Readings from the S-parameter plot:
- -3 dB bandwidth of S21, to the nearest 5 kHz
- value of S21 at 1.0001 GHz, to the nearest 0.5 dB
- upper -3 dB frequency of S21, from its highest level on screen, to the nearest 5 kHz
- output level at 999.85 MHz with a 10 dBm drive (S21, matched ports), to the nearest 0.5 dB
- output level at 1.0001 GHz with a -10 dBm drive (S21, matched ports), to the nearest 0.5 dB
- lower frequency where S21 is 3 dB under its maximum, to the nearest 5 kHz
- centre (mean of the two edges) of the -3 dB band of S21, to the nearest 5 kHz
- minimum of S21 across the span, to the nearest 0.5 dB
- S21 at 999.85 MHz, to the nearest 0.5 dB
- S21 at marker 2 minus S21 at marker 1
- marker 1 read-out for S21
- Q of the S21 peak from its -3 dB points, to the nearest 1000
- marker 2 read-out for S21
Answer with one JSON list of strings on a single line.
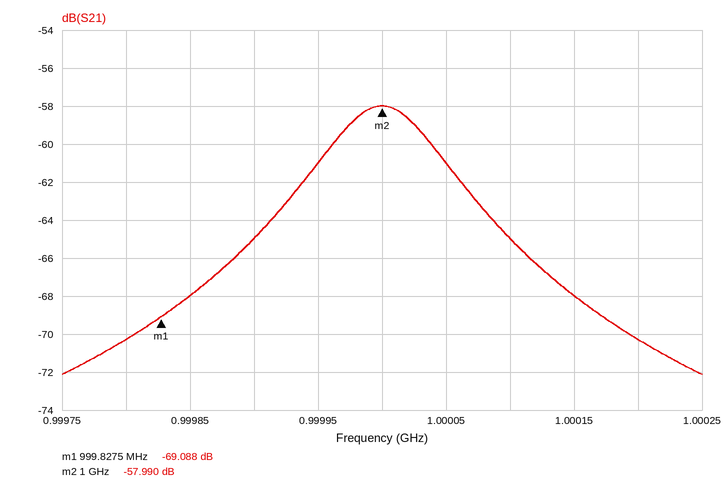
["100 kHz", "-65.0 dB", "1.000050 GHz", "-58.0 dBm", "-75.0 dBm", "999.950 MHz", "1.000000 GHz", "-72.0 dB", "-68.0 dB", "11.098 dB", "-69.088 dB", "10000", "-57.990 dB"]
